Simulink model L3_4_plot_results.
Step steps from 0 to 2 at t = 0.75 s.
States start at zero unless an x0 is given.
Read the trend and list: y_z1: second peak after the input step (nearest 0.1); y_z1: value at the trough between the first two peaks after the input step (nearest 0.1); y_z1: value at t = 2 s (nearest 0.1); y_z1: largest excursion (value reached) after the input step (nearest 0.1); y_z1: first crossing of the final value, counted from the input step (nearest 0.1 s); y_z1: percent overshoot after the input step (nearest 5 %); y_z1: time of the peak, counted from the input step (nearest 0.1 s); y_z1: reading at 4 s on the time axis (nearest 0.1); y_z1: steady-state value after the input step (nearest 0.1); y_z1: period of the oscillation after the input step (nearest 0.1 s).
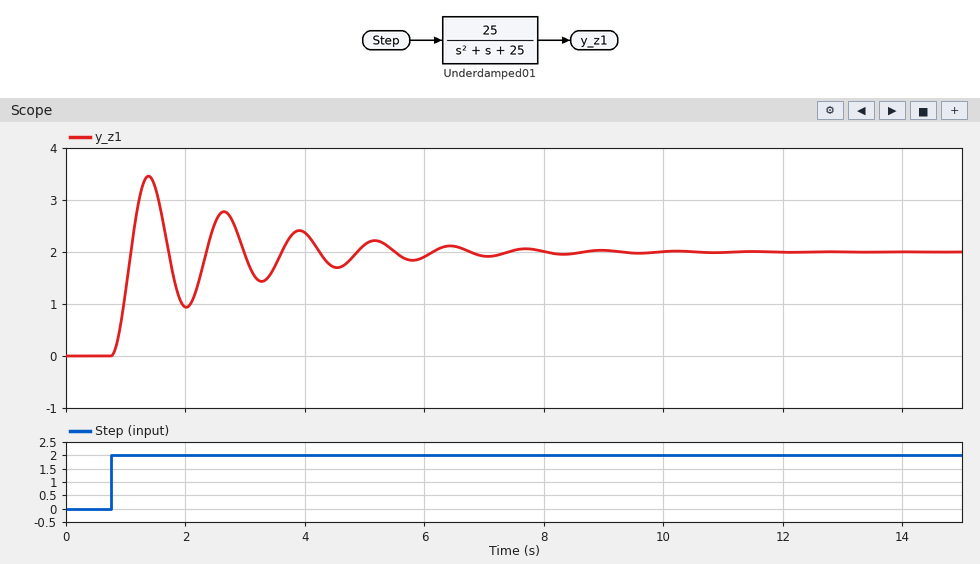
2.8
0.9
0.9
3.5
0.3 s
75 %
0.6 s
2.4
2.0
1.3 s
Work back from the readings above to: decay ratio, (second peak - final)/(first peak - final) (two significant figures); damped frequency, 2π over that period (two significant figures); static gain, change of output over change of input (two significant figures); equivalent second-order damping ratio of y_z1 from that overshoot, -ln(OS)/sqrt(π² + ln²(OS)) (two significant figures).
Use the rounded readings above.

0.53
4.8 rad/s
1.0
0.091
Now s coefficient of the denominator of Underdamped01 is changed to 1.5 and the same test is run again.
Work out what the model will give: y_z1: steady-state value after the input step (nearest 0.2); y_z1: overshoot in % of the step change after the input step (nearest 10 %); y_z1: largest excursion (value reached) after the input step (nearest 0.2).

2.0
60 %
3.2
